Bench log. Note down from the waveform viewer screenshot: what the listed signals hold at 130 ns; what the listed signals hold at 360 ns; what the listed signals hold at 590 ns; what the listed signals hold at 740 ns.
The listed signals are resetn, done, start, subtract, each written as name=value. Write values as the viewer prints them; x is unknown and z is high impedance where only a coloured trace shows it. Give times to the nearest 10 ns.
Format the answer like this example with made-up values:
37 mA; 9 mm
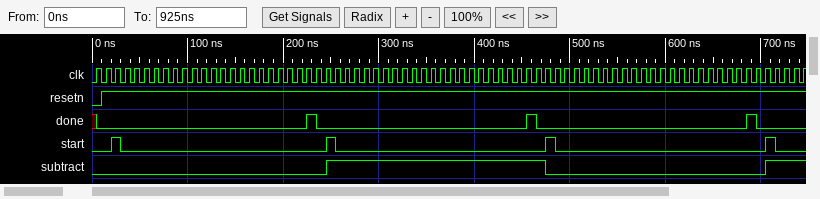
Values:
resetn=1, done=0, start=0, subtract=0; resetn=1, done=0, start=0, subtract=1; resetn=1, done=0, start=0, subtract=0; resetn=1, done=0, start=0, subtract=1
